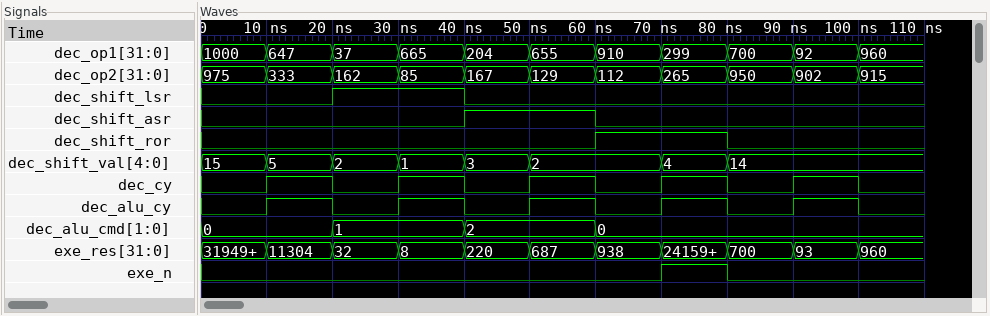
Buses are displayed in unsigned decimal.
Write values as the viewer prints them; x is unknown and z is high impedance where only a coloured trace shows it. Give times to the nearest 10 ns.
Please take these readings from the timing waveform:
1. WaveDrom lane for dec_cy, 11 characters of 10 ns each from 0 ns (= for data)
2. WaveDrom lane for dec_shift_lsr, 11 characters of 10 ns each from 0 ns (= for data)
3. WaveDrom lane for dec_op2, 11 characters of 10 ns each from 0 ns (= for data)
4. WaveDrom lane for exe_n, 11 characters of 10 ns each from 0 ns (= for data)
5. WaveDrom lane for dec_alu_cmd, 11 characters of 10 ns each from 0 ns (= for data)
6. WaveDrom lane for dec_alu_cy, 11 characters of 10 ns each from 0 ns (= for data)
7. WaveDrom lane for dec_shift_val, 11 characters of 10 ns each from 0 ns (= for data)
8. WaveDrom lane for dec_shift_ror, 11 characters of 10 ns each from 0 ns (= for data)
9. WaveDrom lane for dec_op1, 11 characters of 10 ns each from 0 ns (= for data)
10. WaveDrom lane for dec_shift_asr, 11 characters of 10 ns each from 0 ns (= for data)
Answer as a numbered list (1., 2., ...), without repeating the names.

1. {name: 'dec_cy', wave: '01010101010'}
2. {name: 'dec_shift_lsr', wave: '0.1.0......'}
3. {name: 'dec_op2', wave: '===========', data: '975 333 162 85 167 129 112 265 950 902 915'}
4. {name: 'exe_n', wave: '0......10..'}
5. {name: 'dec_alu_cmd', wave: '=.=.=.=....', data: '0 1 2 0'}
6. {name: 'dec_alu_cy', wave: '01010101010'}
7. {name: 'dec_shift_val', wave: '======.==..', data: '15 5 2 1 3 2 4 14'}
8. {name: 'dec_shift_ror', wave: '0.....1.0..'}
9. {name: 'dec_op1', wave: '===========', data: '1000 647 37 665 204 655 910 299 700 92 960'}
10. {name: 'dec_shift_asr', wave: '0...1.0....'}
